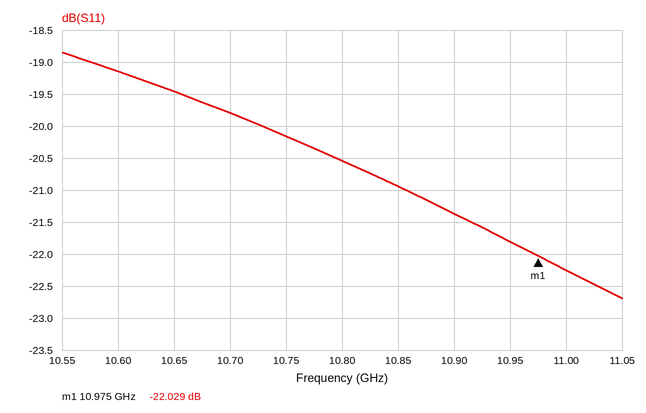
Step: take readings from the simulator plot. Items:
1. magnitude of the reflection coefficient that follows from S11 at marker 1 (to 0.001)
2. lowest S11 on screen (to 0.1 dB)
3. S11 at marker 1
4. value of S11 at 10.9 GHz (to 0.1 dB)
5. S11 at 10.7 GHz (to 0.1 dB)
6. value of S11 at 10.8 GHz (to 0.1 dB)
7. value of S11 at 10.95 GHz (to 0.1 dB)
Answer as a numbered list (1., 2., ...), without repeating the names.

1. 0.079
2. -22.7 dB
3. -22.029 dB
4. -21.4 dB
5. -19.8 dB
6. -20.5 dB
7. -21.8 dB
